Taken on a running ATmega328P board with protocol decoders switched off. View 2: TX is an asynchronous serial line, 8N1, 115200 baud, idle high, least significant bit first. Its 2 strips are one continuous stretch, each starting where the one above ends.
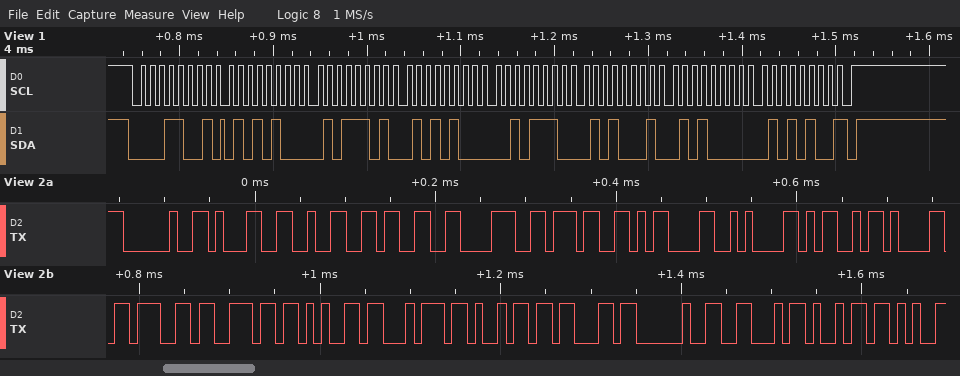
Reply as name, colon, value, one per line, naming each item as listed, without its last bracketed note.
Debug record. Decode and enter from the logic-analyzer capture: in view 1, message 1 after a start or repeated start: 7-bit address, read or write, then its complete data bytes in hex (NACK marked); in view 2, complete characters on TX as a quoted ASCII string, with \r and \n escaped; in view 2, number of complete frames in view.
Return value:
in view 1, message 1 after a start or repeated start: 7-bit address, read or write, then its complete data bytes in hex: 0x0C read: 54 5D 54 2E 51 50 54 NACK
in view 2, complete characters on TX as a quoted ASCII string, with \r and \n escaped: " 12387\r\nMagnetic Fi"
in view 2, number of complete frames in view: 19
